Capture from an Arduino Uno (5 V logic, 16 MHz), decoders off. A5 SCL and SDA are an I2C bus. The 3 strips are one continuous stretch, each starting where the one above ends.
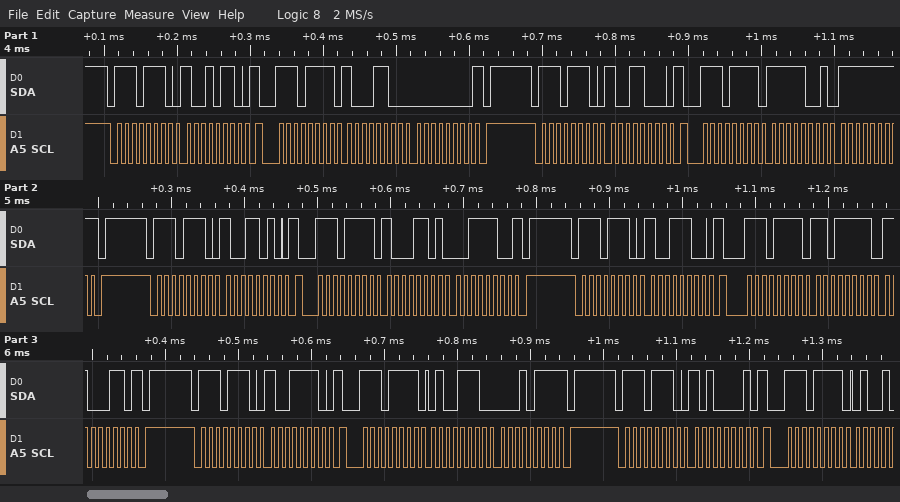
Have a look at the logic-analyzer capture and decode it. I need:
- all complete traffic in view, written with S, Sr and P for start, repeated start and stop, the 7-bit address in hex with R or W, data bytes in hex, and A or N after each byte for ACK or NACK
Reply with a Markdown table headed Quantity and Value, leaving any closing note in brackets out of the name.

| Quantity | Value |
|---|---|
| all complete traffic in view, written with S, Sr and P for start, repeated start and stop, the 7-bit address in hex with R or W, data bytes in hex, and A or N after each byte for ACK or NACK | S 77W A 96 A Sr 77R A 8C A 00 N P S 77W A 98 A Sr 77R A F9 A FF N P S 77W A 9A A Sr 77R A 8D A 3C N P S 77W A 9C A Sr 77R A DF A C6 N P S 77W A 9E A Sr 77R A 4E A 17 N P S 77W A A1 A Sr 77R A |
